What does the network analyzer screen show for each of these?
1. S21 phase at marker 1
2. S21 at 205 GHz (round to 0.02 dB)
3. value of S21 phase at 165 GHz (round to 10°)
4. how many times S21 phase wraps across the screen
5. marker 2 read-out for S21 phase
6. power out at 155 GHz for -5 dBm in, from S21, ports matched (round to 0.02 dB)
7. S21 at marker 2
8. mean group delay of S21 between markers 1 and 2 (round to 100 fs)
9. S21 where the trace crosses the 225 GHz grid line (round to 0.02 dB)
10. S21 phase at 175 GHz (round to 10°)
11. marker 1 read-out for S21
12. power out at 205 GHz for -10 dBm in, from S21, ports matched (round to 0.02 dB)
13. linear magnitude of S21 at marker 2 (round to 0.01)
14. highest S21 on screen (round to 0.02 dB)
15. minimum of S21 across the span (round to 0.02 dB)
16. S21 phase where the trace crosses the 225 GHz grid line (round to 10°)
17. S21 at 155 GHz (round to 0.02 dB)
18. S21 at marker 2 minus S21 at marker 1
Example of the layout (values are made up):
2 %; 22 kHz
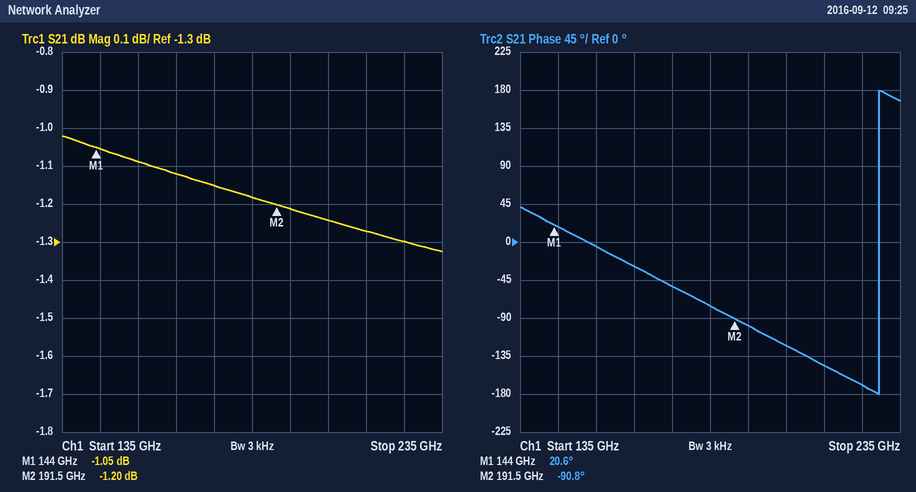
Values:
20.6°; -1.24 dB; -30°; 1; -90.8°; -6.08 dBm; -1.20 dB; 6.5 ps; -1.30 dB; -50°; -1.05 dB; -11.24 dBm; 0.87; -1.02 dB; -1.32 dB; -170°; -1.08 dB; -0.15 dB
